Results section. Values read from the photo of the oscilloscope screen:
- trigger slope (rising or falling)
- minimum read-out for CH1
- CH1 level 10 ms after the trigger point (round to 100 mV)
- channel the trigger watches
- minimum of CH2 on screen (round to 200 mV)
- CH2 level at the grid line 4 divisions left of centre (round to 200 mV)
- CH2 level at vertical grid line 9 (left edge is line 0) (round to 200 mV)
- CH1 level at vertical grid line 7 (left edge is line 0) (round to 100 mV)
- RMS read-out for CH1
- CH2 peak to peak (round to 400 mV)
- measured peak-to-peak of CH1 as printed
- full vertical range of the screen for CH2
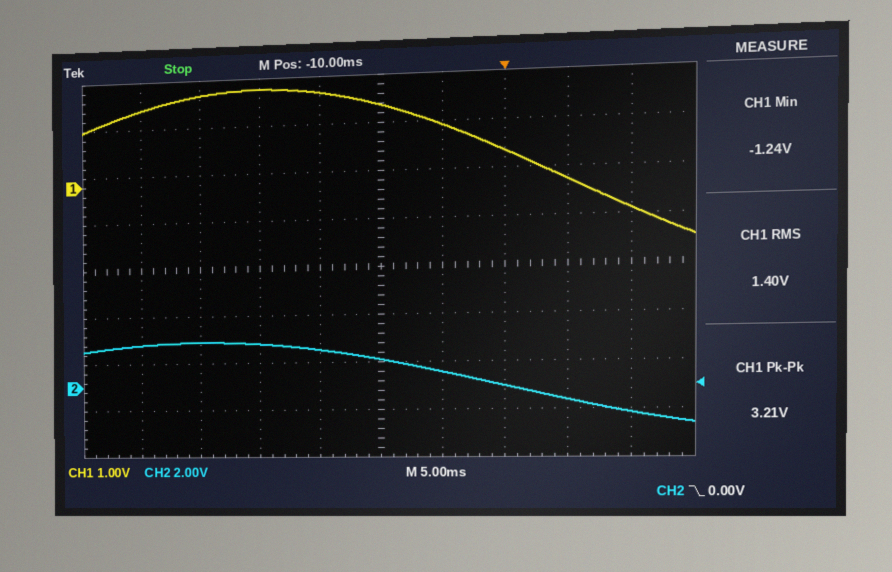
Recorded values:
falling
-1.24 V
-700 mV
CH2
-1.6 V
1.8 V
-1.2 V
600 mV
1.40 V
3.6 V
3.21 V
16 V
